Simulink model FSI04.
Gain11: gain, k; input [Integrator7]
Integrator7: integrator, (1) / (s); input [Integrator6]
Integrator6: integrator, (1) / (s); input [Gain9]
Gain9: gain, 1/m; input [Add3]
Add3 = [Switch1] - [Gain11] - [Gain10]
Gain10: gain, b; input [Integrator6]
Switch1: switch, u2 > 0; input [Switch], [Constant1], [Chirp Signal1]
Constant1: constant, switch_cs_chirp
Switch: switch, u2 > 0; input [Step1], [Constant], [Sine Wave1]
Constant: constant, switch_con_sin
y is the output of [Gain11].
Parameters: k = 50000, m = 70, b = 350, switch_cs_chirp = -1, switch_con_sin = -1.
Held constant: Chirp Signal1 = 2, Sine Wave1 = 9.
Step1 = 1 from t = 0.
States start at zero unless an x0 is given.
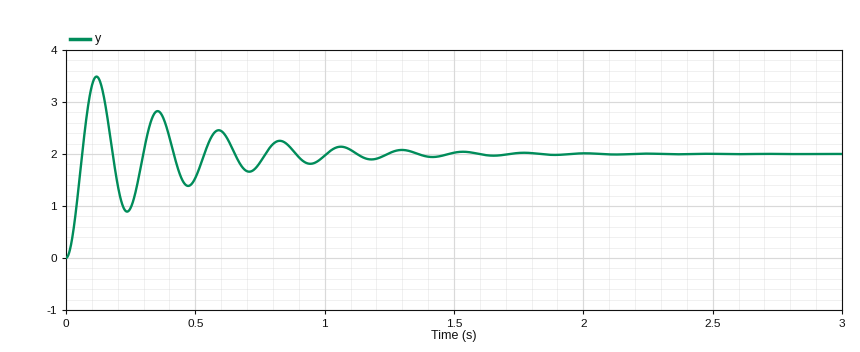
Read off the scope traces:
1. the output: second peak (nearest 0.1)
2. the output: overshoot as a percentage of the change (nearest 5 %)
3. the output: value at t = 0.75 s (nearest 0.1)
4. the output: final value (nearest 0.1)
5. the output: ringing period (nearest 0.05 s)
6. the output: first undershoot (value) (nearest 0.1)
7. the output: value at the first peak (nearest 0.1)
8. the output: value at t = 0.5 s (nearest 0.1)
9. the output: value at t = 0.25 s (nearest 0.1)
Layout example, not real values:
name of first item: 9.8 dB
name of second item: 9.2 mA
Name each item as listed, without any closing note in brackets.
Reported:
the output: second peak: 2.8
the output: overshoot as a percentage of the change: 75 %
the output: value at t = 0.75 s: 1.8
the output: final value: 2.0
the output: ringing period: 0.25 s
the output: first undershoot (value): 0.9
the output: value at the first peak: 3.5
the output: value at t = 0.5 s: 1.5
the output: value at t = 0.25 s: 1.0
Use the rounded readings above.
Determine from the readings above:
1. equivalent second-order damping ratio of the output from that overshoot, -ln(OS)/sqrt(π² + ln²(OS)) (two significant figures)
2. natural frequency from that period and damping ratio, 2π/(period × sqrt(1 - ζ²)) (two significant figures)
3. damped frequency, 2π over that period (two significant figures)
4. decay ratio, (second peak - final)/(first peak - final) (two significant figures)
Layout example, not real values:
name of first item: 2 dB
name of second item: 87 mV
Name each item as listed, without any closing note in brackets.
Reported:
equivalent second-order damping ratio of the output from that overshoot, -ln(OS)/sqrt(π² + ln²(OS)): 0.091
natural frequency from that period and damping ratio, 2π/(period × sqrt(1 - ζ²)): 25 rad/s
damped frequency, 2π over that period: 25 rad/s
decay ratio, (second peak - final)/(first peak - final): 0.53
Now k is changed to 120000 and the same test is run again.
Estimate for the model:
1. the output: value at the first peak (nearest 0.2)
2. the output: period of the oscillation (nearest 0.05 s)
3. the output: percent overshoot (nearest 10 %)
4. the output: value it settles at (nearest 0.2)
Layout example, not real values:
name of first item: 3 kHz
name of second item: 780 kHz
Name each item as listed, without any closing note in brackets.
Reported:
the output: value at the first peak: 3.6
the output: period of the oscillation: 0.15 s
the output: percent overshoot: 80 %
the output: value it settles at: 2.0
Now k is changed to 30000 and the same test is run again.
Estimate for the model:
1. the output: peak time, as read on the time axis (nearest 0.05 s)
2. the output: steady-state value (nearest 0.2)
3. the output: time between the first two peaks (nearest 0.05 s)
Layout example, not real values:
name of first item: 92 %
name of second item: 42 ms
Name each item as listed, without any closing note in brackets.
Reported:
the output: peak time, as read on the time axis: 0.15 s
the output: steady-state value: 2.0
the output: time between the first two peaks: 0.30 s
